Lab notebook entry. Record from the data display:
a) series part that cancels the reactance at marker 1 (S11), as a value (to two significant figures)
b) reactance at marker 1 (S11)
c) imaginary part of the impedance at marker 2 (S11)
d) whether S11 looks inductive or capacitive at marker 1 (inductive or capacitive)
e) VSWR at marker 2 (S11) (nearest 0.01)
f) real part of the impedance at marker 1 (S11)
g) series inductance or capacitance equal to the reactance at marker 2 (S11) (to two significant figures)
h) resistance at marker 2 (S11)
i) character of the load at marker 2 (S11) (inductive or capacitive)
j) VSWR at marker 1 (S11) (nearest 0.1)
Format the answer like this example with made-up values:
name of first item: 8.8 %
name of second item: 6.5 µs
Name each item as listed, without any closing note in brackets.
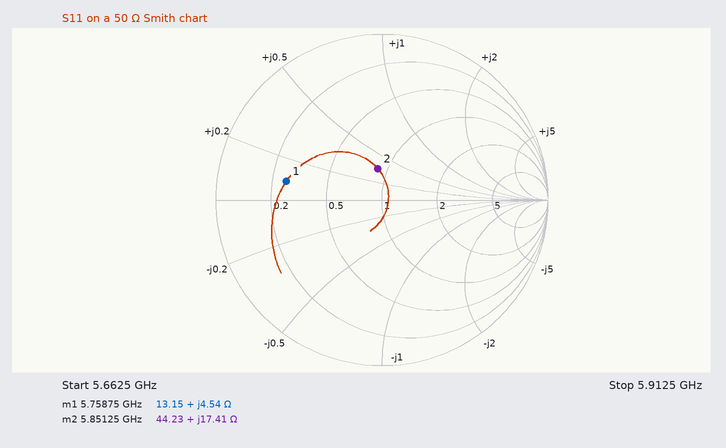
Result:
series part that cancels the reactance at marker 1 (S11), as a value: 6.1 pF
reactance at marker 1: +4.54 Ω
imaginary part of the impedance at marker 2: +17.41 Ω
whether S11 looks inductive or capacitive at marker 1: inductive
VSWR at marker 2 (S11): 1.47
real part of the impedance at marker 1: 13.15 Ω
series inductance or capacitance equal to the reactance at marker 2 (S11): 470 pH
resistance at marker 2: 44.23 Ω
character of the load at marker 2 (S11): inductive
VSWR at marker 1 (S11): 3.8
